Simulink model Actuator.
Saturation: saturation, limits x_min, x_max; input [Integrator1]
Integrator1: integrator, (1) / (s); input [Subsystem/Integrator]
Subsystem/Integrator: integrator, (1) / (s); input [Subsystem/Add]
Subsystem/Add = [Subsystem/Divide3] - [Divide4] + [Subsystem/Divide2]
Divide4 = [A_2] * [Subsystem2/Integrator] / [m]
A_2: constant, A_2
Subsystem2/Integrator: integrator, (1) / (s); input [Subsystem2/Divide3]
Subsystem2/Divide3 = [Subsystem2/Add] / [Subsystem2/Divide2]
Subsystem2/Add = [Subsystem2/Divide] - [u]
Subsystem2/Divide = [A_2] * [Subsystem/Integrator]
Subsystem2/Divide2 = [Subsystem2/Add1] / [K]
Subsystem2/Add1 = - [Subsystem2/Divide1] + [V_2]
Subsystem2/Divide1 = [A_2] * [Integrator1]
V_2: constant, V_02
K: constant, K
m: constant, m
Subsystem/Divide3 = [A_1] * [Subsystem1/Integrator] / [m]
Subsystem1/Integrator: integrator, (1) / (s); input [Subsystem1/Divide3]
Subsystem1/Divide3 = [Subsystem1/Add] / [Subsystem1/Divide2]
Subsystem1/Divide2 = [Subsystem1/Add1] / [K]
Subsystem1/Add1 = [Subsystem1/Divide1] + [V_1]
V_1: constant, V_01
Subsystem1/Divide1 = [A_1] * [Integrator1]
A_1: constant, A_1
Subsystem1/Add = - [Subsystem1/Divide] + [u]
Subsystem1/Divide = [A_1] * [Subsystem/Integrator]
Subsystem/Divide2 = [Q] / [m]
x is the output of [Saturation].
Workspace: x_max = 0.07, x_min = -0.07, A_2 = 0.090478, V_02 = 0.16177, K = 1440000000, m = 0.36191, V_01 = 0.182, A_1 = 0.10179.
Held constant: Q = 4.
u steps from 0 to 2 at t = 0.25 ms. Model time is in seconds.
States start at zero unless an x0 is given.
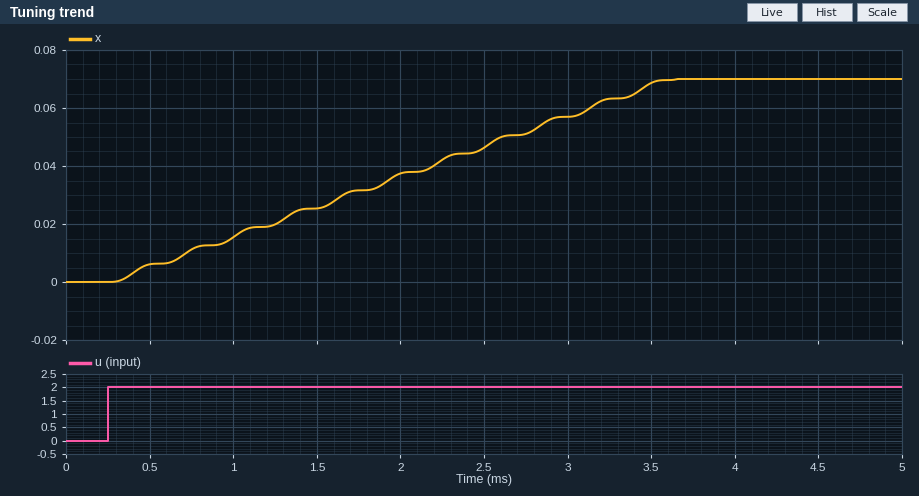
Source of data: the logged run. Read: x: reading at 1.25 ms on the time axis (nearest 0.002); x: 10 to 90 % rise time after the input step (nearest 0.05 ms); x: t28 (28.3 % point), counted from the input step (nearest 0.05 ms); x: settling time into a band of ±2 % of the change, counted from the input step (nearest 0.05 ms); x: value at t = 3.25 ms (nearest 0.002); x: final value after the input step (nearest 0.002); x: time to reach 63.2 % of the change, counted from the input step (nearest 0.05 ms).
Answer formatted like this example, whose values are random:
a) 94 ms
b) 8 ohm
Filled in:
a) 0.020
b) 2.60 ms
c) 1.00 ms
d) 3.25 ms
e) 0.064
f) 0.070
g) 2.10 ms
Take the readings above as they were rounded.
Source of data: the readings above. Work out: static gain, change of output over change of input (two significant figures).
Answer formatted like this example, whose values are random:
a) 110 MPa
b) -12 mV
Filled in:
a) 0.035
